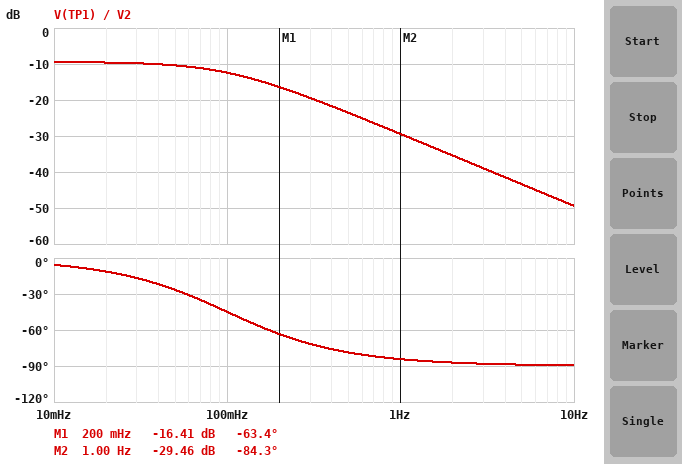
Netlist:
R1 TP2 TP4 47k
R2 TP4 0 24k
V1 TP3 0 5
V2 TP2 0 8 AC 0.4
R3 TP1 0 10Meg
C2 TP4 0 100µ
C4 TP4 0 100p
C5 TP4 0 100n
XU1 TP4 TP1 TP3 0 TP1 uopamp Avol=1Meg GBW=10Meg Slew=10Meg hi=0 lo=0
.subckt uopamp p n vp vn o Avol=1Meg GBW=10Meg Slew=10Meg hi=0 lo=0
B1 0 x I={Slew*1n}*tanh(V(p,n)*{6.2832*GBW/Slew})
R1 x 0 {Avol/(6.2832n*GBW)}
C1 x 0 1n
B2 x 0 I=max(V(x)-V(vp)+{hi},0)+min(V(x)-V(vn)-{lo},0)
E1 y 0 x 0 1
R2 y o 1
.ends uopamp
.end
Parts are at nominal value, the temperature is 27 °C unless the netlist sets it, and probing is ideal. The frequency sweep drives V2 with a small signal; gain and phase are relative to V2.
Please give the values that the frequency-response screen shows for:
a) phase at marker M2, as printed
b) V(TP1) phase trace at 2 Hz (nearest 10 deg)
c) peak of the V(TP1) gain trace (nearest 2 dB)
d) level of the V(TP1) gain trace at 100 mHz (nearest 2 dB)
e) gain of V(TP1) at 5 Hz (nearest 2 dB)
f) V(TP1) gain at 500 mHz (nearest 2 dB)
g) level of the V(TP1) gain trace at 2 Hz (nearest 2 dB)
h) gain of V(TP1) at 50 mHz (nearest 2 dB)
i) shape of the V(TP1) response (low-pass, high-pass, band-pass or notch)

-84.3 deg
-90 deg
-10 dB
-12 dB
-44 dB
-24 dB
-36 dB
-10 dB
low-pass
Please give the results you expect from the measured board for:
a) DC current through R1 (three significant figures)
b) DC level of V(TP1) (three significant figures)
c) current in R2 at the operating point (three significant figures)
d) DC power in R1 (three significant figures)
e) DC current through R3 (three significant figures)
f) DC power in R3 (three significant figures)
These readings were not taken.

113 µA
2.70 V
113 µA
597 µW
270 nA
731 nW
